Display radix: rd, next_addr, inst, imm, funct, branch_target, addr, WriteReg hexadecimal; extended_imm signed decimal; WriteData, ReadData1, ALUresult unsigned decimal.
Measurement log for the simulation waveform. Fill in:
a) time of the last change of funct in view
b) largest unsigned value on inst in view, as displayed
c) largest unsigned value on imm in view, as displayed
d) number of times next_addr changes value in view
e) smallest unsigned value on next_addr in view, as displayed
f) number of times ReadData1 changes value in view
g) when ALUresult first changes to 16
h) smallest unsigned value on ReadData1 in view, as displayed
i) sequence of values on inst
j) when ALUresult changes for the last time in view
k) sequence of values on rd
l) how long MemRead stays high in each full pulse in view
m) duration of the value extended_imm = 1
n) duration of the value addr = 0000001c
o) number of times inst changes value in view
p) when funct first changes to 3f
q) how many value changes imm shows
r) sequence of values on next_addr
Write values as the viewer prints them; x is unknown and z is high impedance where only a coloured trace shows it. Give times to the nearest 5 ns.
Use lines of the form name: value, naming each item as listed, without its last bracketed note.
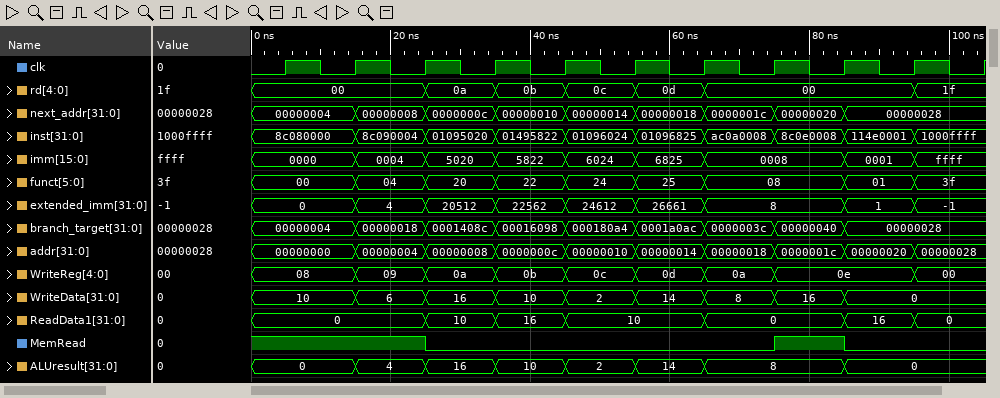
time of the last change of funct in view: 95 ns
largest unsigned value on inst in view, as displayed: ac0a0008
largest unsigned value on imm in view, as displayed: ffff
number of times next_addr changes value in view: 8
smallest unsigned value on next_addr in view, as displayed: 00000004
number of times ReadData1 changes value in view: 6
when ALUresult first changes to 16: 25 ns
smallest unsigned value on ReadData1 in view, as displayed: 0
sequence of values on inst: 8c080000, 8c090004, 01095020, 01495822, 01096024, 01096825, ac0a0008, 8c0e0008, 114e0001, 1000ffff
when ALUresult changes for the last time in view: 85 ns
sequence of values on rd: 00, 0a, 0b, 0c, 0d, 00, 1f
how long MemRead stays high in each full pulse in view: 10 ns
duration of the value extended_imm = 1: 10 ns
duration of the value addr = 0000001c: 10 ns
number of times inst changes value in view: 9
when funct first changes to 3f: 95 ns
how many value changes imm shows: 8
sequence of values on next_addr: 00000004, 00000008, 0000000c, 00000010, 00000014, 00000018, 0000001c, 00000020, 00000028
